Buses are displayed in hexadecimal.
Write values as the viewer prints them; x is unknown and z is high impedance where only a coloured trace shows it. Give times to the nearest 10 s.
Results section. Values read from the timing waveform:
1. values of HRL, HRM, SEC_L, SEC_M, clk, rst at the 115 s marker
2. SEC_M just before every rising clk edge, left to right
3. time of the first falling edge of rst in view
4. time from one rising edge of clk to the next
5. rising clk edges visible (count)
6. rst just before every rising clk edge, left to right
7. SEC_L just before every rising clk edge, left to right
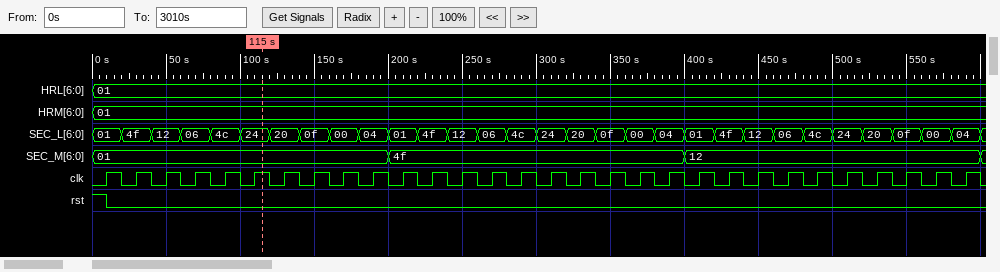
HRL=01, HRM=01, SEC_L=24, SEC_M=01, clk=1, rst=0
01, 01, 01, 01, 01, 01, 01, 01, 01, 01, 4f, 4f, 4f, 4f, 4f, 4f, 4f, 4f, 4f, 4f, 12, 12, 12, 12, 12, 12, 12, 12, 12, 12
10 s
20 s
30
1 0 0 0 0 0 0 0 0 0 0 0 0 0 0 0 0 0 0 0 0 0 0 0 0 0 0 0 0 0
01, 4f, 12, 06, 4c, 24, 20, 0f, 00, 04, 01, 4f, 12, 06, 4c, 24, 20, 0f, 00, 04, 01, 4f, 12, 06, 4c, 24, 20, 0f, 00, 04
